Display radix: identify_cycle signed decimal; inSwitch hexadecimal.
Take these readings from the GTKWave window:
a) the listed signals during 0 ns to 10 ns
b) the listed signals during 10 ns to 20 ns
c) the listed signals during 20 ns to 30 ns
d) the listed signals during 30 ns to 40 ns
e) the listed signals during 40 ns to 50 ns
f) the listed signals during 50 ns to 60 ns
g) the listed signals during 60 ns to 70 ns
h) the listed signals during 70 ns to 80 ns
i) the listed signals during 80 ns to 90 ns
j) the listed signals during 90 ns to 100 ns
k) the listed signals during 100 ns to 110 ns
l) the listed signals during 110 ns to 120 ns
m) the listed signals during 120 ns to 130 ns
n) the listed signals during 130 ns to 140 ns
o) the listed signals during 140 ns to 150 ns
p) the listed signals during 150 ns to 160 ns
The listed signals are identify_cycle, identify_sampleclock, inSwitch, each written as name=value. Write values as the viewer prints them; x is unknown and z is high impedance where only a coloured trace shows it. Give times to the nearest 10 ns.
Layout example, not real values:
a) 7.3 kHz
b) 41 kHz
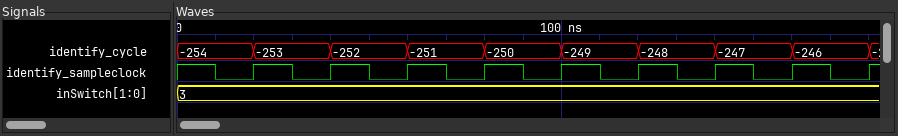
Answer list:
a) identify_cycle=-254, identify_sampleclock=1, inSwitch=3
b) identify_cycle=-254, identify_sampleclock=0, inSwitch=3
c) identify_cycle=-253, identify_sampleclock=1, inSwitch=3
d) identify_cycle=-253, identify_sampleclock=0, inSwitch=3
e) identify_cycle=-252, identify_sampleclock=1, inSwitch=3
f) identify_cycle=-252, identify_sampleclock=0, inSwitch=3
g) identify_cycle=-251, identify_sampleclock=1, inSwitch=3
h) identify_cycle=-251, identify_sampleclock=0, inSwitch=3
i) identify_cycle=-250, identify_sampleclock=1, inSwitch=3
j) identify_cycle=-250, identify_sampleclock=0, inSwitch=3
k) identify_cycle=-249, identify_sampleclock=1, inSwitch=3
l) identify_cycle=-249, identify_sampleclock=0, inSwitch=3
m) identify_cycle=-248, identify_sampleclock=1, inSwitch=3
n) identify_cycle=-248, identify_sampleclock=0, inSwitch=3
o) identify_cycle=-247, identify_sampleclock=1, inSwitch=3
p) identify_cycle=-247, identify_sampleclock=0, inSwitch=3
